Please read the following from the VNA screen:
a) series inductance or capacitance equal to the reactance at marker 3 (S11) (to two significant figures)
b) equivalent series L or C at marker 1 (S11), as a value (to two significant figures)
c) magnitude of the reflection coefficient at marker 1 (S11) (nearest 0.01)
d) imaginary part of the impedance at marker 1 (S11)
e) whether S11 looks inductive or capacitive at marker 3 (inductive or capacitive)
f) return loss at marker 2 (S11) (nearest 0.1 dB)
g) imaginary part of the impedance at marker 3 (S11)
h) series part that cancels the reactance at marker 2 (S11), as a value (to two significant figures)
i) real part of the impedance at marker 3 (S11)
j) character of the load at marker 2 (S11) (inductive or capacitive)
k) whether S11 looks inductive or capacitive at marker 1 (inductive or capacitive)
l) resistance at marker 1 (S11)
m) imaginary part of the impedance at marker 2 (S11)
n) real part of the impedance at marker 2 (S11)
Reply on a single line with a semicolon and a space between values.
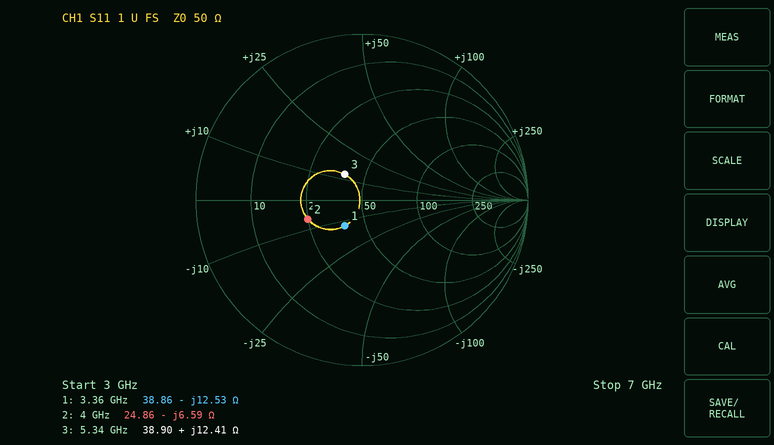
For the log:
370 pH; 3.8 pF; 0.19; -12.53 Ω; inductive; 9.2 dB; +12.41 Ω; 260 pH; 38.90 Ω; capacitive; capacitive; 38.86 Ω; -6.59 Ω; 24.86 Ω
